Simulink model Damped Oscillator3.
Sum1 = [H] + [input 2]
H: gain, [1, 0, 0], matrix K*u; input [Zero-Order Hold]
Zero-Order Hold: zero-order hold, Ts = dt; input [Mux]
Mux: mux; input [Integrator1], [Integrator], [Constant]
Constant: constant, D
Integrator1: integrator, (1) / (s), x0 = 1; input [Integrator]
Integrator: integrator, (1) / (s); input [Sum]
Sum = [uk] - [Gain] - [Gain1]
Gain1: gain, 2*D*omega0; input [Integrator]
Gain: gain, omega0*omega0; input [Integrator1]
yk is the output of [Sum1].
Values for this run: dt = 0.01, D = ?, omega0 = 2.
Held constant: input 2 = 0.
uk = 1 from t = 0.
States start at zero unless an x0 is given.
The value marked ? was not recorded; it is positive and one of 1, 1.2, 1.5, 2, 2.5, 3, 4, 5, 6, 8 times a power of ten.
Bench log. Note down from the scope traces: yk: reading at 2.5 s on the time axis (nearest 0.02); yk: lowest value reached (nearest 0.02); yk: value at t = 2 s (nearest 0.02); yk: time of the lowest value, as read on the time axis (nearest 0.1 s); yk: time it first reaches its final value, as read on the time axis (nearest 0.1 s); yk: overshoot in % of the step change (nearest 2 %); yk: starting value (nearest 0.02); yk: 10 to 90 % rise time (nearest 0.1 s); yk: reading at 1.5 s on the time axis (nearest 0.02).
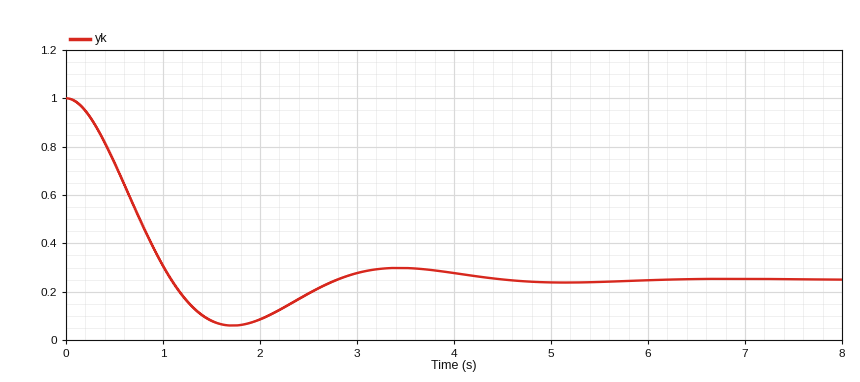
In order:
0.20
0.06
0.08
1.7 s
1.1 s
26 %
1.00
0.7 s
0.08
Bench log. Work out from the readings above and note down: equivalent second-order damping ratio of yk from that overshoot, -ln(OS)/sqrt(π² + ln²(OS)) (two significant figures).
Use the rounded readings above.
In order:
0.39
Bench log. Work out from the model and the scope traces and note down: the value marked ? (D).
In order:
0.4
